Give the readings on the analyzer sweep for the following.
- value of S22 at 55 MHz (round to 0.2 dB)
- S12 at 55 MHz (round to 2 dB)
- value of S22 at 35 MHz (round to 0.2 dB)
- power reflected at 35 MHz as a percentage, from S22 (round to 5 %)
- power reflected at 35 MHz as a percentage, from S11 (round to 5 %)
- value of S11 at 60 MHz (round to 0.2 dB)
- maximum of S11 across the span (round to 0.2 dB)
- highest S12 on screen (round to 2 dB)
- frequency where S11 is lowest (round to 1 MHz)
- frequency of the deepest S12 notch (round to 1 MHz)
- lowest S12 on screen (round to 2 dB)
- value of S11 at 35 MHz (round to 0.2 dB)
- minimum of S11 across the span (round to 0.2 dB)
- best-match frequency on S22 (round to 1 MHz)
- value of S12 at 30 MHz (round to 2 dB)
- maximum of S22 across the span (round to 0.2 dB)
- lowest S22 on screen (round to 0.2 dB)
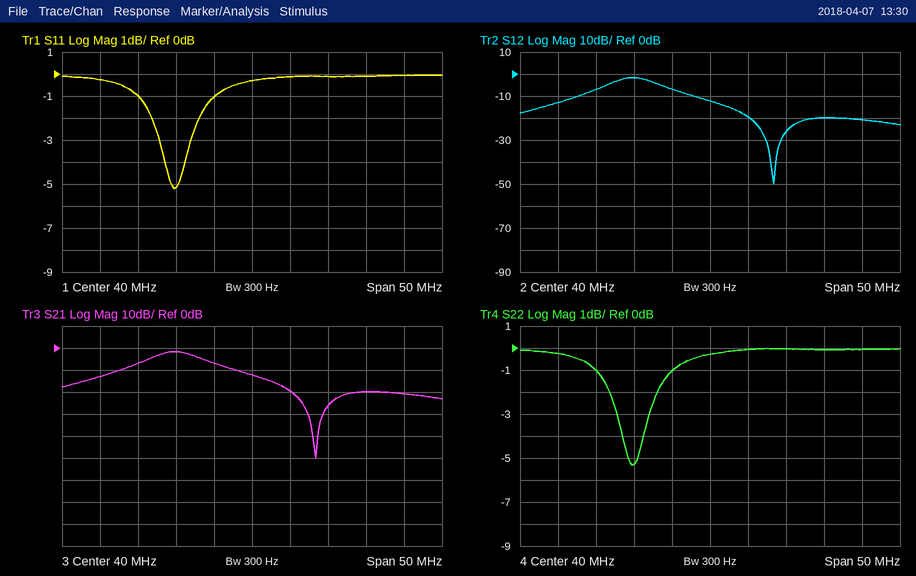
0.0 dB
-20 dB
-1.0 dB
80 %
80 %
0.0 dB
0.0 dB
-2 dB
30 MHz
48 MHz
-50 dB
-1.0 dB
-5.2 dB
30 MHz
-2 dB
0.0 dB
-5.4 dB
